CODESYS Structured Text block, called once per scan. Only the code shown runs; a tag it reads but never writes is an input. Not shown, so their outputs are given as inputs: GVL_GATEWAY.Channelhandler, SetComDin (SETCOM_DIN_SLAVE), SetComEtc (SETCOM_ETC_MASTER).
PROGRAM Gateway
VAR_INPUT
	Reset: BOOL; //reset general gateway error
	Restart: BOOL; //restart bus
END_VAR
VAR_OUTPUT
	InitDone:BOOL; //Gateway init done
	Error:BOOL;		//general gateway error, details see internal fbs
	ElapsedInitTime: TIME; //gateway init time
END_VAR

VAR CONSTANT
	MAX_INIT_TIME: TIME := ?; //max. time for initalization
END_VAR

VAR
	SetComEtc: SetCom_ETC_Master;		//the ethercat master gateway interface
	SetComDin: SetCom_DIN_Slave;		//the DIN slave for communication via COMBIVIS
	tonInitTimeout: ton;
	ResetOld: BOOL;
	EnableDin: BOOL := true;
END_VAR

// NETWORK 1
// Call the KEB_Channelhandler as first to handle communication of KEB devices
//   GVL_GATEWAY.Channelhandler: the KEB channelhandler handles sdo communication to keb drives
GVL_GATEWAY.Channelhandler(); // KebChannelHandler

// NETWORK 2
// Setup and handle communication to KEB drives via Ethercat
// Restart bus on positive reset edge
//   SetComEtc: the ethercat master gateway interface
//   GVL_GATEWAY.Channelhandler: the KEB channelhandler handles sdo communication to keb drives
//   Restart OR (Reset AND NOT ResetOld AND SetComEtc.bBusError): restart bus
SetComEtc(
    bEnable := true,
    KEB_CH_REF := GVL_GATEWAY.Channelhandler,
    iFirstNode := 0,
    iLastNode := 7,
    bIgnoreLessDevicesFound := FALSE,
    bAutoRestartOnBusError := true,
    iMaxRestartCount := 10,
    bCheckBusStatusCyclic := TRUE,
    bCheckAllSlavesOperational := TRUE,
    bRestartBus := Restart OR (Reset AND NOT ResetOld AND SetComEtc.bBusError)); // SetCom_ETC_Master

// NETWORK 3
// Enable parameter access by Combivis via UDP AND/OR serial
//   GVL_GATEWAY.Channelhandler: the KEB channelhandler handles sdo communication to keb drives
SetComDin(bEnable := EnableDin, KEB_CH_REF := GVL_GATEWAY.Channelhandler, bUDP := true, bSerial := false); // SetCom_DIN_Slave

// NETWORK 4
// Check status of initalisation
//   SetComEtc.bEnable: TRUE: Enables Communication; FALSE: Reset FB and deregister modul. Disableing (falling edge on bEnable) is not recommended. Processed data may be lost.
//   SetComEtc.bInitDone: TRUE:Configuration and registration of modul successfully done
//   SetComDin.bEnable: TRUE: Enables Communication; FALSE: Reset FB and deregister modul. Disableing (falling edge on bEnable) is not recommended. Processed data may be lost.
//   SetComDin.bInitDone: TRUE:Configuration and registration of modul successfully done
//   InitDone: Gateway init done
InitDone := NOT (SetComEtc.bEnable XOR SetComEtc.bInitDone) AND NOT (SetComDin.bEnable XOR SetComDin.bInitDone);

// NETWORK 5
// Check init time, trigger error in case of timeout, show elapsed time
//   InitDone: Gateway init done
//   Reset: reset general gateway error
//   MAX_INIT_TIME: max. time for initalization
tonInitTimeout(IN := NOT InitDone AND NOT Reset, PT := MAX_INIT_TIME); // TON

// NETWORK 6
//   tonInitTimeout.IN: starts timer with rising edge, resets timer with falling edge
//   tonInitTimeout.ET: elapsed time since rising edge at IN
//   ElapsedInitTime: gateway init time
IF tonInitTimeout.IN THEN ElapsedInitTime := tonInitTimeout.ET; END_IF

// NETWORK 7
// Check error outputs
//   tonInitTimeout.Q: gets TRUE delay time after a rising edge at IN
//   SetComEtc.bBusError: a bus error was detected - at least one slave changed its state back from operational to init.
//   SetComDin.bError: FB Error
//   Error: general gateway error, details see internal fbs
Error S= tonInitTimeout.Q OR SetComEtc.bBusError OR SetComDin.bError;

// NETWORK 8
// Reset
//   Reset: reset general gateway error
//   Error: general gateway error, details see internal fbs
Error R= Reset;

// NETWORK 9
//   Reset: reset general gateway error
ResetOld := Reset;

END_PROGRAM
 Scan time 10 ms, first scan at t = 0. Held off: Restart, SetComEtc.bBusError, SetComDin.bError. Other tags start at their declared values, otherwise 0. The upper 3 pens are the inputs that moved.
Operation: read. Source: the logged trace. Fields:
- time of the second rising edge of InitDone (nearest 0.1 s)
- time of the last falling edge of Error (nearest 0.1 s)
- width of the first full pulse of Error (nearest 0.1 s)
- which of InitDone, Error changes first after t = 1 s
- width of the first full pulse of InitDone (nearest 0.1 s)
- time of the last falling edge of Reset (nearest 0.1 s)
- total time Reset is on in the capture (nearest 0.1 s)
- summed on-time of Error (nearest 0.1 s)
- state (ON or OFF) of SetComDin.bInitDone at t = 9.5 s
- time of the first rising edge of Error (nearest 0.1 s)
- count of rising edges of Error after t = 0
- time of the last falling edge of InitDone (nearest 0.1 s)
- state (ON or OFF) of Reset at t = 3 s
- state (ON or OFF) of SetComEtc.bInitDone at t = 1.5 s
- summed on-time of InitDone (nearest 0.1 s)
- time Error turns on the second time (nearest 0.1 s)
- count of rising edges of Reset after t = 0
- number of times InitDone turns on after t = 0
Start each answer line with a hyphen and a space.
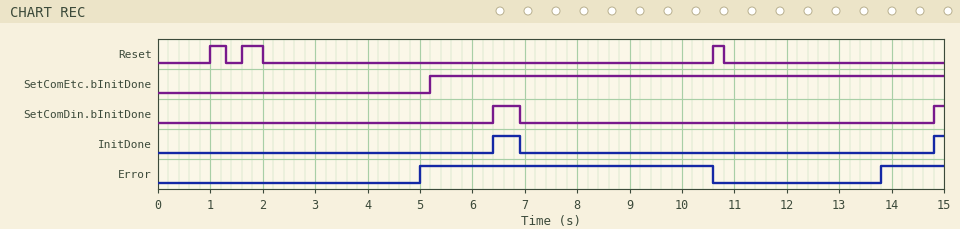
- 14.8 s
- 10.6 s
- 5.6 s
- Error
- 0.5 s
- 10.8 s
- 0.9 s
- 6.8 s
- OFF
- 5.0 s
- 2
- 6.9 s
- OFF
- OFF
- 0.7 s
- 13.8 s
- 3
- 2
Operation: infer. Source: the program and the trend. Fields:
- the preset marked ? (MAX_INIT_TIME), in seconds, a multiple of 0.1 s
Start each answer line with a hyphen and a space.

- 3.0 s
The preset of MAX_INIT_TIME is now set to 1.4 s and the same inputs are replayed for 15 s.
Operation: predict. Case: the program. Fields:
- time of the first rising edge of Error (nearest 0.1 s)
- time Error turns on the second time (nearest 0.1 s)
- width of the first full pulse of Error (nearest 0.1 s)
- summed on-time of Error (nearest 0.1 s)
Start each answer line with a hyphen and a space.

- 3.4 s
- 12.2 s
- 7.2 s
- 10.0 s
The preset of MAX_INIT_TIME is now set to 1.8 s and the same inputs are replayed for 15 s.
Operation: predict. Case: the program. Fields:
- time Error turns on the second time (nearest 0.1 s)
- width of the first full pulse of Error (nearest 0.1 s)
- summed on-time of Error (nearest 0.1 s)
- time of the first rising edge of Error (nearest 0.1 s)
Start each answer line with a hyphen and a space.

- 12.6 s
- 6.8 s
- 9.2 s
- 3.8 s
